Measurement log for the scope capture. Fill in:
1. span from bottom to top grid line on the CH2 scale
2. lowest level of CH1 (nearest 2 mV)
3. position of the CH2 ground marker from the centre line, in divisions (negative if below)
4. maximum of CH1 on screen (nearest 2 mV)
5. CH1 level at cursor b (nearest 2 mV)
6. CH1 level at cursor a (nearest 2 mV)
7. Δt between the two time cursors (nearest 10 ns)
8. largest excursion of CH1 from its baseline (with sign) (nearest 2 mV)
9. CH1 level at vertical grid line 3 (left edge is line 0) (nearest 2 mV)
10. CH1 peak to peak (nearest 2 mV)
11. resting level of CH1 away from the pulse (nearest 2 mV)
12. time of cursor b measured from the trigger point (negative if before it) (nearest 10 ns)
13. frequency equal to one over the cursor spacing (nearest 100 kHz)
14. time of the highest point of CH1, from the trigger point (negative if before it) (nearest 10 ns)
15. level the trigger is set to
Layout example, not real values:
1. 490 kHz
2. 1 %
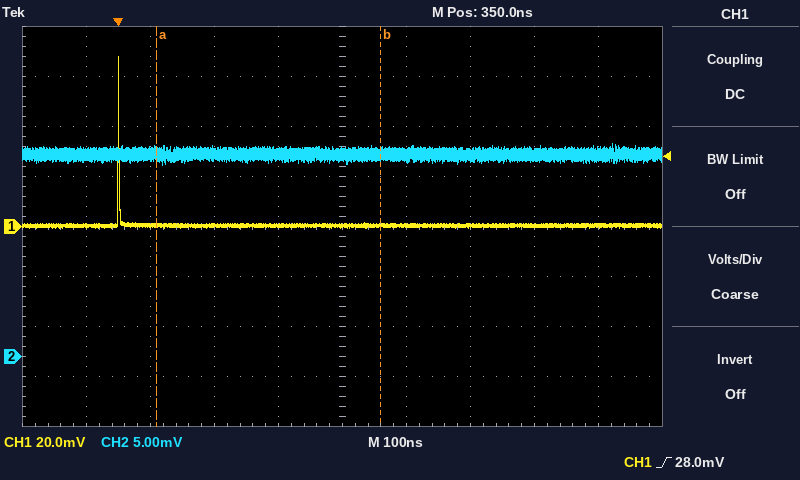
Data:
1. 40 mV
2. 0 mV
3. -2.6 div
4. 68 mV
5. 0 mV
6. 0 mV
7. 350 ns
8. +68 mV
9. 0 mV
10. 68 mV
11. 0 mV
12. +410 ns
13. 2.9 MHz
14. 0 ns
15. 28.0 mV
